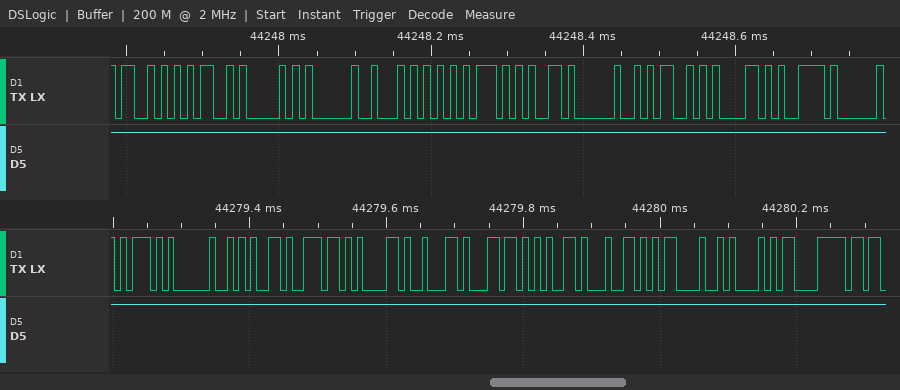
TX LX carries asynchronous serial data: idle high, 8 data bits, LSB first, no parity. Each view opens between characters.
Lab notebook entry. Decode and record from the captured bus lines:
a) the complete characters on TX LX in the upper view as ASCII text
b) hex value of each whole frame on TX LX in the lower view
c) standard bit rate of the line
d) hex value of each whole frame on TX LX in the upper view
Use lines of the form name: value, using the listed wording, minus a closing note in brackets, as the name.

the complete characters on TX LX in the upper view as ASCII text: "SMP Tue May"
hex value of each whole frame on TX LX in the lower view: 5D, 20, 65, 6E, 61, 62, 6C, 65, 64, 0D, 0A, 0D
standard bit rate of the line: 115200 baud
hex value of each whole frame on TX LX in the upper view: 53, 4D, 50, 20, 54, 75, 65, 20, 4D, 61, 79
